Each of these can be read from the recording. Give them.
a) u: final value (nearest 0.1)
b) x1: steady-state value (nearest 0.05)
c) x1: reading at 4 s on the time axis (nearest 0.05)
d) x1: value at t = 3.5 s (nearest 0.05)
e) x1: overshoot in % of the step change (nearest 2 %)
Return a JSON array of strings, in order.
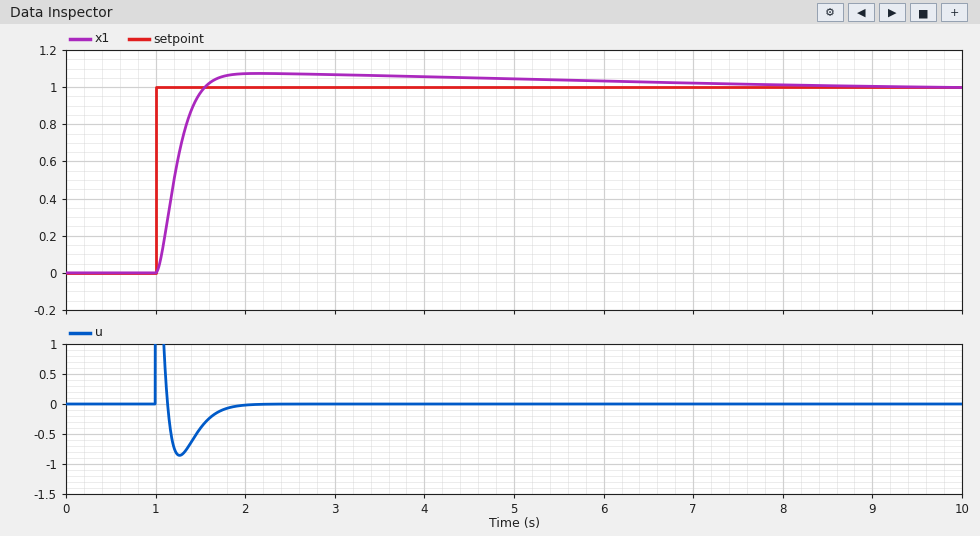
["0.0", "1.00", "1.05", "1.05", "8 %"]
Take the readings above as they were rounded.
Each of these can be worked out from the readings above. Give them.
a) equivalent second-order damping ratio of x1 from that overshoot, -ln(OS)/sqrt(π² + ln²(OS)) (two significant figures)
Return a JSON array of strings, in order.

["0.63"]
